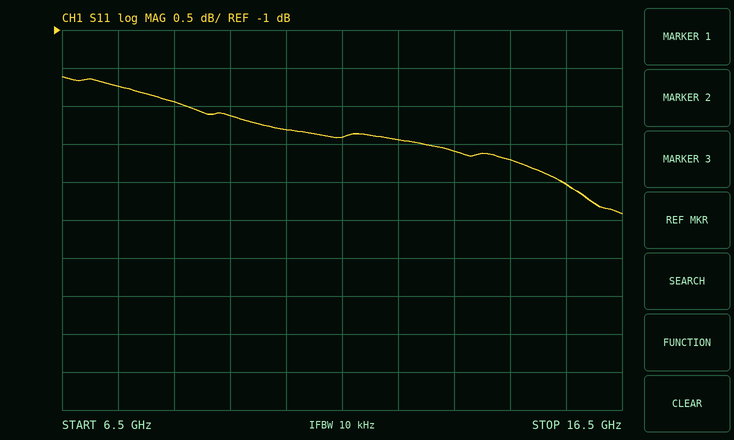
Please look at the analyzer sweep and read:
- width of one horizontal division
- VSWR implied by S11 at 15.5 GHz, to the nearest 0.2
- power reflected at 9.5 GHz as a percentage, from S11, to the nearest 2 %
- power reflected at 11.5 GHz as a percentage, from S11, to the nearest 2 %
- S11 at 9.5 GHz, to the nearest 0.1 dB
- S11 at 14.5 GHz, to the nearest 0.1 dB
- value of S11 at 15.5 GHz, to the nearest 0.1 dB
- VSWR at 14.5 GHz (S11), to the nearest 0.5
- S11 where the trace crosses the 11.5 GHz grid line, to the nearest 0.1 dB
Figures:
1 GHz
5.8
62 %
58 %
-2.1 dB
-2.7 dB
-3.0 dB
6.5
-2.4 dB
